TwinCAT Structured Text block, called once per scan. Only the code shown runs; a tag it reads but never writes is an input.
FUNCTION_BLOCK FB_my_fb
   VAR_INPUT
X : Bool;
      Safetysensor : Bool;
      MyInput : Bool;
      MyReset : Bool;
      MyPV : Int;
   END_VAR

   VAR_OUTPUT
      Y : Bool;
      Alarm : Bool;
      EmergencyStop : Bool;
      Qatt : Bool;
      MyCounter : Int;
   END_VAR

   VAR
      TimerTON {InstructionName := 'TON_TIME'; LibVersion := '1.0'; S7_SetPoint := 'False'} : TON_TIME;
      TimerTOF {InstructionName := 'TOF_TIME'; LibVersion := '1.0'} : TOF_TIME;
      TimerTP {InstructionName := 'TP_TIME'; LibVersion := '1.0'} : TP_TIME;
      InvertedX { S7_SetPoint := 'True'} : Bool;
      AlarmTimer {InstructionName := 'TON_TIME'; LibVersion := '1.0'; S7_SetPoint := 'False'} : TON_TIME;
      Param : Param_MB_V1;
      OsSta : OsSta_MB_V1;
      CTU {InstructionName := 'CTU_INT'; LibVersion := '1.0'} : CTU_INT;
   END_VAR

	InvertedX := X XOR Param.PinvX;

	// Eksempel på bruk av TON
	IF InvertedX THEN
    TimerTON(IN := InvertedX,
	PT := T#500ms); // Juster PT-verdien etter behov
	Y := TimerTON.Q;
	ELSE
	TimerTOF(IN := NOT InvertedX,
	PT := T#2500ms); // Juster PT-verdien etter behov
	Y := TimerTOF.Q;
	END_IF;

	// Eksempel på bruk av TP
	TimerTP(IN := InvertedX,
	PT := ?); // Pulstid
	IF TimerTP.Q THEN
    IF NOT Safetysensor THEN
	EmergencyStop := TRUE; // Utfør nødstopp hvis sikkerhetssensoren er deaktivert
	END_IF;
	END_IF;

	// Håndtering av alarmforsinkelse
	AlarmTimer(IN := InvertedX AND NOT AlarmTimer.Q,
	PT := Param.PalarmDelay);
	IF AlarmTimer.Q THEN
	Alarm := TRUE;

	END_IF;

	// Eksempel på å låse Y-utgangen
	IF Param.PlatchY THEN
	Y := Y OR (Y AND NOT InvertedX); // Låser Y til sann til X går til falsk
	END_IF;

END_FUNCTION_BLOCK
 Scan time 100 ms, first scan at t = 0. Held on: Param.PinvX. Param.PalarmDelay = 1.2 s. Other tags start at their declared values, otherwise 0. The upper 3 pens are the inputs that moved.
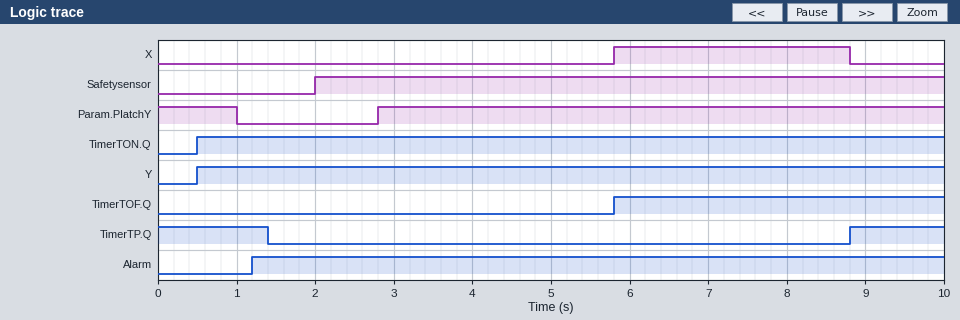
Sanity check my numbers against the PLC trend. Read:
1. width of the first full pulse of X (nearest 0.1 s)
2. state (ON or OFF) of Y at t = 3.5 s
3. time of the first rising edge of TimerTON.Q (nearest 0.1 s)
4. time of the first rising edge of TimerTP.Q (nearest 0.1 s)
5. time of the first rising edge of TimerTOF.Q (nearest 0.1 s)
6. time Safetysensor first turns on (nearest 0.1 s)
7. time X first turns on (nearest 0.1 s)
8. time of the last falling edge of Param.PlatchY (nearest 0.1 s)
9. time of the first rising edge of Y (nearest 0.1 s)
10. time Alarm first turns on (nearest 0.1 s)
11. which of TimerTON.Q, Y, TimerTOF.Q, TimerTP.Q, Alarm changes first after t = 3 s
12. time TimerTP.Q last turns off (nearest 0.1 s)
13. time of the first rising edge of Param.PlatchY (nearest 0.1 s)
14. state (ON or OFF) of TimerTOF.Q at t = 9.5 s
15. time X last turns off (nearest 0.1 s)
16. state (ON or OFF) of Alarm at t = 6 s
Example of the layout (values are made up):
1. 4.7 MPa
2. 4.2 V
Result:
1. 3.0 s
2. ON
3. 0.5 s
4. 8.8 s
5. 5.8 s
6. 2.0 s
7. 5.8 s
8. 1.0 s
9. 0.5 s
10. 1.2 s
11. TimerTOF.Q
12. 1.4 s
13. 2.8 s
14. ON
15. 8.8 s
16. ON
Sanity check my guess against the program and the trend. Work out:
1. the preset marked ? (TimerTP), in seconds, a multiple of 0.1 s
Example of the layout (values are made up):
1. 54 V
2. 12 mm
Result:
1. 1.4 s
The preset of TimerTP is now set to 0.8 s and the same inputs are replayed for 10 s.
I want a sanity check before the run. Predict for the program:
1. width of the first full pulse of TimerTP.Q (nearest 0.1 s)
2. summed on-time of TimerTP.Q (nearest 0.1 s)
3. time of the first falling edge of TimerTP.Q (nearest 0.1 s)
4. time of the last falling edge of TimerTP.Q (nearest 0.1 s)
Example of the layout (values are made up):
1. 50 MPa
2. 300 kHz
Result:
1. 0.8 s
2. 1.6 s
3. 0.8 s
4. 9.6 s
